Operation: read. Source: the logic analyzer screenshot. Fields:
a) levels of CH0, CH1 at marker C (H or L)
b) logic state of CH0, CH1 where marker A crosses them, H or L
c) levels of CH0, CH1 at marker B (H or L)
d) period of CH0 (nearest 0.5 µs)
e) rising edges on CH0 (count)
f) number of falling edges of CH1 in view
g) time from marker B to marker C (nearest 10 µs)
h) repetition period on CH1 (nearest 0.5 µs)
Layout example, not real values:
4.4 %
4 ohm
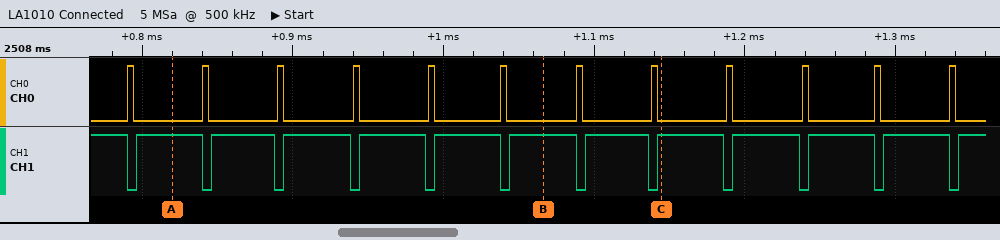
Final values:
CH0=L, CH1=H
CH0=L, CH1=H
CH0=L, CH1=H
49.5 µs
12
12
80 µs
49.5 µs
